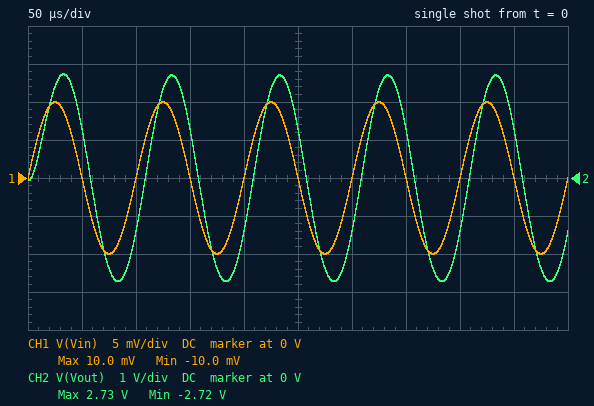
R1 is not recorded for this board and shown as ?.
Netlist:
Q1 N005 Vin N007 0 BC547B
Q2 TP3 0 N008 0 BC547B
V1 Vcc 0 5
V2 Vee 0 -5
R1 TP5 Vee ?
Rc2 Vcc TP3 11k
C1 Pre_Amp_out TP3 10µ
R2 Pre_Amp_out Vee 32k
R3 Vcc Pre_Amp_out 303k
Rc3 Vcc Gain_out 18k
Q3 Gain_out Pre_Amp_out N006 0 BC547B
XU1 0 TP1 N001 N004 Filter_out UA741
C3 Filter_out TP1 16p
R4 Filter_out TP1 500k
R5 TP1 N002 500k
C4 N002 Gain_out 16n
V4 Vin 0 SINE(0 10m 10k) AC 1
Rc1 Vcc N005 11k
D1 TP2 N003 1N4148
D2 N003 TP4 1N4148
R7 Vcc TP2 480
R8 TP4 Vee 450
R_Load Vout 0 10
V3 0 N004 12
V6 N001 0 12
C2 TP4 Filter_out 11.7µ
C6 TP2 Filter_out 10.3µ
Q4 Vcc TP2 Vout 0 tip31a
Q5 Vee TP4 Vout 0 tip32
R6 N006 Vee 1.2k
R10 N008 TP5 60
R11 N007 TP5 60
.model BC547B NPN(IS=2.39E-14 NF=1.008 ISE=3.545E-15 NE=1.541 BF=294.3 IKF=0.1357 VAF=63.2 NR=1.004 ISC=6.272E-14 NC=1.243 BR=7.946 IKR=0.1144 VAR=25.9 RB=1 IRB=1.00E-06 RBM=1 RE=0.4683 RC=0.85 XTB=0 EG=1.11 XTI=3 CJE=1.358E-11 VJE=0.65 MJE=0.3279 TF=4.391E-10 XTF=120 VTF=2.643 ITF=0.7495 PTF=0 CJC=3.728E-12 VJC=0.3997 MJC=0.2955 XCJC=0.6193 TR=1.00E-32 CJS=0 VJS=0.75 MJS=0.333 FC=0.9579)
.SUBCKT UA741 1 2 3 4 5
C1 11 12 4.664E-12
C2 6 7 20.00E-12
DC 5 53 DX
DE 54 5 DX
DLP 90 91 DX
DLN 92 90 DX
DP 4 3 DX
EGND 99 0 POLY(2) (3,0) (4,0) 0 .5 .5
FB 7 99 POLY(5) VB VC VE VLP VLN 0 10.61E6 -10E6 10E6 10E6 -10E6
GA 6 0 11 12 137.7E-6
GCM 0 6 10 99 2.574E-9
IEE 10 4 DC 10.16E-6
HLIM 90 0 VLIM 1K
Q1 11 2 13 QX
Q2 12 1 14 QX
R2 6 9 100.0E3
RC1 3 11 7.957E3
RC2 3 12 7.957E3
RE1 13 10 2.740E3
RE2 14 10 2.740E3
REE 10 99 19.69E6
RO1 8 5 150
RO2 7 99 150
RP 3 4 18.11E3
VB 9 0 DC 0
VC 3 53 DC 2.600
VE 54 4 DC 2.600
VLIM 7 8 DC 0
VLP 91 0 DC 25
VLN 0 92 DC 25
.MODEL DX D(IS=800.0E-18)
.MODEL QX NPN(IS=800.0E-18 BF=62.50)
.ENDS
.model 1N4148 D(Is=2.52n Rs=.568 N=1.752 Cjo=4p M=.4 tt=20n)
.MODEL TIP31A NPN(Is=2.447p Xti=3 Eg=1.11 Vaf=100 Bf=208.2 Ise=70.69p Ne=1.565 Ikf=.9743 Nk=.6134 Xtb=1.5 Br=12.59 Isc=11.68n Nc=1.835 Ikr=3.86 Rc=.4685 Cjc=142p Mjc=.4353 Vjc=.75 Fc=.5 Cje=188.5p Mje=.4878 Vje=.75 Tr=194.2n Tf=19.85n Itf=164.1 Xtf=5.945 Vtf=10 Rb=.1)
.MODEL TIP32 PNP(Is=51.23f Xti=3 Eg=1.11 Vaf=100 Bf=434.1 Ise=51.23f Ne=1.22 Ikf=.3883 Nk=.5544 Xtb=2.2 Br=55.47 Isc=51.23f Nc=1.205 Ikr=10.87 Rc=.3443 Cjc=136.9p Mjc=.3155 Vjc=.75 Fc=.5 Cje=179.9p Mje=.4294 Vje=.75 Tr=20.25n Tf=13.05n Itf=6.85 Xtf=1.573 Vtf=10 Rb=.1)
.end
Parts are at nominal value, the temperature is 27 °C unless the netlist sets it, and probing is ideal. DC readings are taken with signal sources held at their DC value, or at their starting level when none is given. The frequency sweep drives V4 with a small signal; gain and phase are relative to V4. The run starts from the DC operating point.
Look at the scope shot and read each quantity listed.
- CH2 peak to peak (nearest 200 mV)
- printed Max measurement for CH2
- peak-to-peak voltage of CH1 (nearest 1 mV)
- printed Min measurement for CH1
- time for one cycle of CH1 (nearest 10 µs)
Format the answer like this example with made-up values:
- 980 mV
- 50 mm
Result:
- 5.4 V
- 2.73 V
- 20 mV
- -10.0 mV
- 100 µs
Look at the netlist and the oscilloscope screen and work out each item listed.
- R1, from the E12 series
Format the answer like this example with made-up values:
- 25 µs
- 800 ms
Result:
- 8.2 kΩ
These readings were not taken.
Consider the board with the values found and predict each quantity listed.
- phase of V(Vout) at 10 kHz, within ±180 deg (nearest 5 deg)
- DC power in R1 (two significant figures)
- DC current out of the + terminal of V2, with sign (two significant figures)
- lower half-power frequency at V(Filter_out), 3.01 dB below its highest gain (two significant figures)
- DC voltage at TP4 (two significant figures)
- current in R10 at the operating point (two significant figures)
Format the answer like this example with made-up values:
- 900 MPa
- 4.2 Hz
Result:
- -30 deg
- 2.3 mW
- -110 mA
- 19 Hz
- -800 mV
- 270 µA
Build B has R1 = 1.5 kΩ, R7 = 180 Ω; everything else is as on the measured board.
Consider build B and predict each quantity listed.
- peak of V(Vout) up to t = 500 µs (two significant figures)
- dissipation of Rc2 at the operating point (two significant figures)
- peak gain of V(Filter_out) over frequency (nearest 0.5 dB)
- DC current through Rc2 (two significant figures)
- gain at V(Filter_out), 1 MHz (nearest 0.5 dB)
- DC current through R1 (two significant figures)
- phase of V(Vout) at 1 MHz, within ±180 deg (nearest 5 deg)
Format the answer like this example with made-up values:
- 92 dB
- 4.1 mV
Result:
- 1.7 V
- 2.9 mW
- 7.0 dB
- 520 µA
- -34.5 dB
- 2.8 mA
- 120 deg
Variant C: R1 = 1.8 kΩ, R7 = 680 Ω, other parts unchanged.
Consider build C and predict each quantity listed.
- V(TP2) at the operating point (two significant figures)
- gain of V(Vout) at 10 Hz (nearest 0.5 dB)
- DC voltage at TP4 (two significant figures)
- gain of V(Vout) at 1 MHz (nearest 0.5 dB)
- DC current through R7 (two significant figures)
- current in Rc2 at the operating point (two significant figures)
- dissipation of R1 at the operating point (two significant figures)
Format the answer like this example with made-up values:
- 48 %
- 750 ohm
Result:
- -32 mV
- -9.5 dB
- -1.4 V
- -29.5 dB
- 7.4 mA
- 520 µA
- 10 mW
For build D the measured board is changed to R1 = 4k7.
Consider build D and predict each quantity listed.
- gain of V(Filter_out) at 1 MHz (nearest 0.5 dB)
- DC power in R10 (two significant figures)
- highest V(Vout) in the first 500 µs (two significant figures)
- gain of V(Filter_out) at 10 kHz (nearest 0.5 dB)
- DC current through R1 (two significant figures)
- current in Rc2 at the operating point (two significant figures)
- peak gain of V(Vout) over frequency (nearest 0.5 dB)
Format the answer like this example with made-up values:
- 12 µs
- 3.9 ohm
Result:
- 7.5 dB
- 13 µW
- 3.6 V
- 51.5 dB
- 930 µA
- 460 µA
- 52.5 dB
